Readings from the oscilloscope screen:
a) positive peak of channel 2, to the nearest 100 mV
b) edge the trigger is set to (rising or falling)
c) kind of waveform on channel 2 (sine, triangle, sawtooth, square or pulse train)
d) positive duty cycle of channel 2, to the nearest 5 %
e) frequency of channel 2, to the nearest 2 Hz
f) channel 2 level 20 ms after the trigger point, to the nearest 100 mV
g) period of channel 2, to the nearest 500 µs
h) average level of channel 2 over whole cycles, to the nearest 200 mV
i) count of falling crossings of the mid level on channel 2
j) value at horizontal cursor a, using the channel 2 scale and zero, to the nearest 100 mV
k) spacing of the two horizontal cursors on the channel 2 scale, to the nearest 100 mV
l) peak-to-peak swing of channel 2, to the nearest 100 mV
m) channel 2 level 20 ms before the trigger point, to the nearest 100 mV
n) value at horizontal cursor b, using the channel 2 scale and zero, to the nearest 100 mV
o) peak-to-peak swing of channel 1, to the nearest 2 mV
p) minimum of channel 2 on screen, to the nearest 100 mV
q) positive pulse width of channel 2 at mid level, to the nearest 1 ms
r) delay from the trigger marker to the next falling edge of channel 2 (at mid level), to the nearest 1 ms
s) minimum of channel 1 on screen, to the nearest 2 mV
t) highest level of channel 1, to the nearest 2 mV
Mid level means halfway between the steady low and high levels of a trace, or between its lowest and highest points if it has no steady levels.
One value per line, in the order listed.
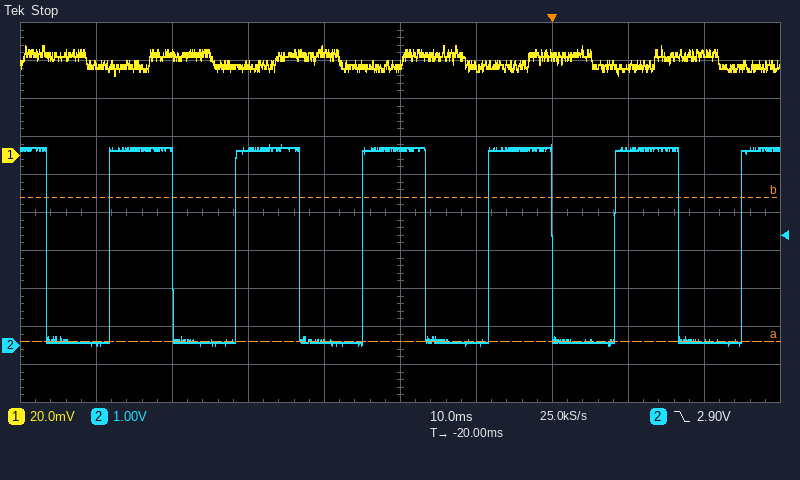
5.3 V
falling
square
50 %
60 Hz
100 mV
16.5 ms
2.6 V
6
100 mV
3.8 V
5.3 V
5.2 V
3.9 V
16 mV
0.0 V
8 ms
17 ms
42 mV
58 mV
